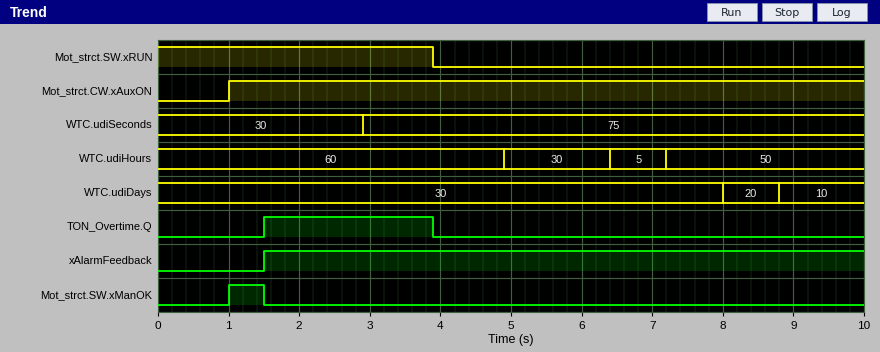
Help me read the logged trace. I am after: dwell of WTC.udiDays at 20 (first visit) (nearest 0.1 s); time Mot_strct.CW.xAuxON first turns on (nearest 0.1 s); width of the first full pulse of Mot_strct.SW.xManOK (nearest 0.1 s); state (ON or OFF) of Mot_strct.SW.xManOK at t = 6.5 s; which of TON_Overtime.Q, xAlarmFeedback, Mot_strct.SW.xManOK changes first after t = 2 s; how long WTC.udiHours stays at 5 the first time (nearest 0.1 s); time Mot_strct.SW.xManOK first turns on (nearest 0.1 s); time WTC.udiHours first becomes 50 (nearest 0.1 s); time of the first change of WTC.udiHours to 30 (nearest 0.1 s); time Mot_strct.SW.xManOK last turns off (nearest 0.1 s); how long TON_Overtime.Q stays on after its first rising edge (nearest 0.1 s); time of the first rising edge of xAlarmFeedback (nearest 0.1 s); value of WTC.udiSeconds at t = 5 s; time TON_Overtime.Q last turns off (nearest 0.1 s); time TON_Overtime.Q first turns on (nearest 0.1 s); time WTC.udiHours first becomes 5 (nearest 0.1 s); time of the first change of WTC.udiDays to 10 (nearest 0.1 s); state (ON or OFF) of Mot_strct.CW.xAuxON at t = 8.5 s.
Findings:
0.8 s
1.0 s
0.5 s
OFF
TON_Overtime.Q
0.8 s
1.0 s
7.2 s
4.9 s
1.5 s
2.4 s
1.5 s
75
3.9 s
1.5 s
6.4 s
8.8 s
ON
